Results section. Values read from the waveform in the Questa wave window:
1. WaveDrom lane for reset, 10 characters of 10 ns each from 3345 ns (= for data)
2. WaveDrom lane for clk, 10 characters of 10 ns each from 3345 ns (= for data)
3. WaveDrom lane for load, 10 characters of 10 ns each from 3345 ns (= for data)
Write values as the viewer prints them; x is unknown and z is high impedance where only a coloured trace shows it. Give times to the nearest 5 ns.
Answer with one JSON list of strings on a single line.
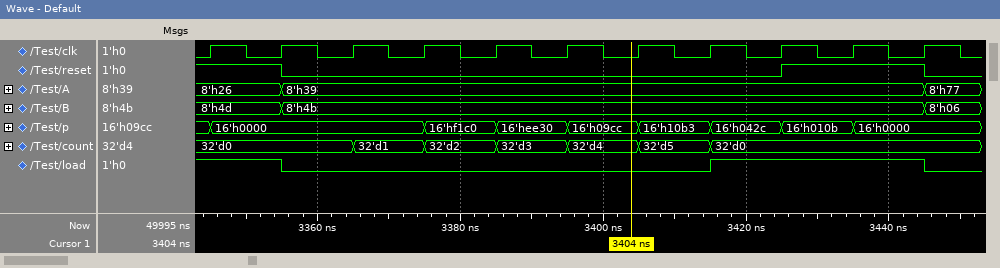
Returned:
["{name: 'reset', wave: '10......1.'}", "{name: 'clk', wave: 'p.........'}", "{name: 'load', wave: '10.....1..'}"]
